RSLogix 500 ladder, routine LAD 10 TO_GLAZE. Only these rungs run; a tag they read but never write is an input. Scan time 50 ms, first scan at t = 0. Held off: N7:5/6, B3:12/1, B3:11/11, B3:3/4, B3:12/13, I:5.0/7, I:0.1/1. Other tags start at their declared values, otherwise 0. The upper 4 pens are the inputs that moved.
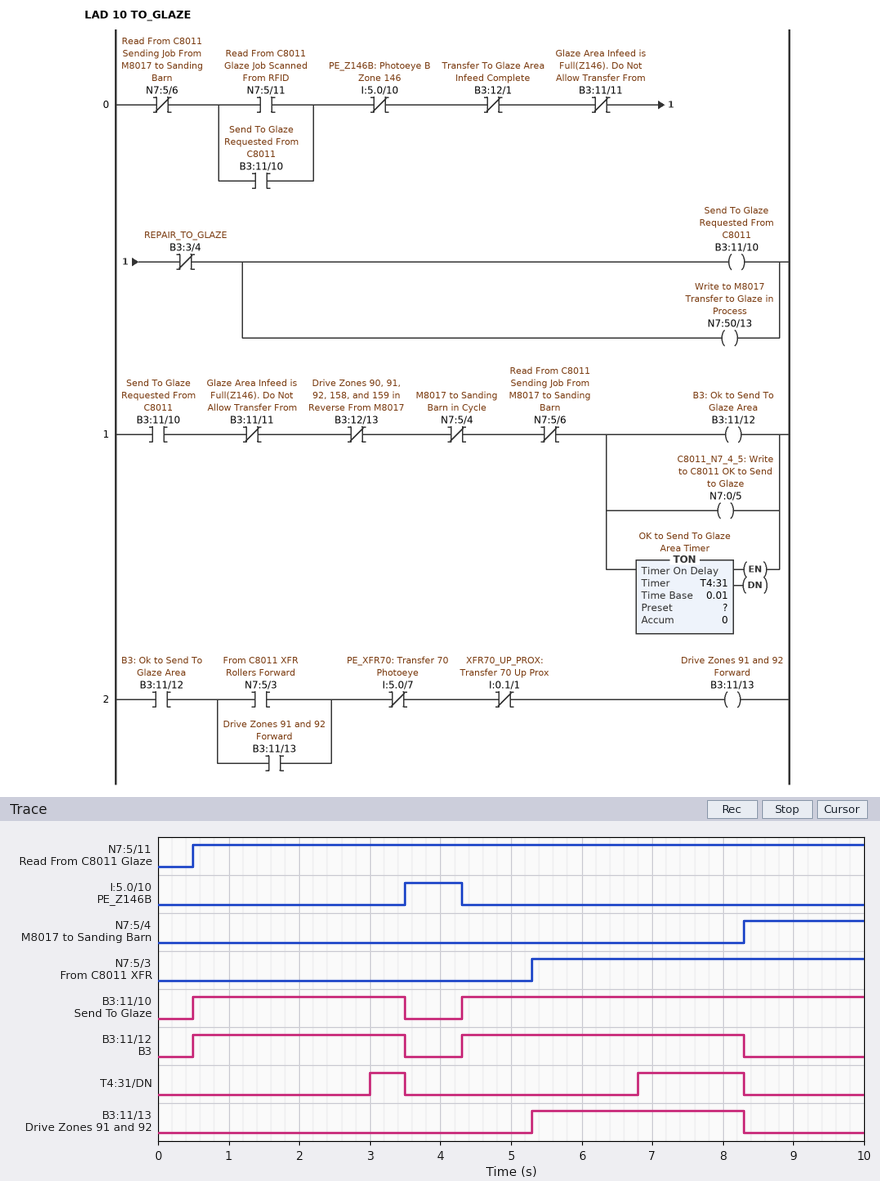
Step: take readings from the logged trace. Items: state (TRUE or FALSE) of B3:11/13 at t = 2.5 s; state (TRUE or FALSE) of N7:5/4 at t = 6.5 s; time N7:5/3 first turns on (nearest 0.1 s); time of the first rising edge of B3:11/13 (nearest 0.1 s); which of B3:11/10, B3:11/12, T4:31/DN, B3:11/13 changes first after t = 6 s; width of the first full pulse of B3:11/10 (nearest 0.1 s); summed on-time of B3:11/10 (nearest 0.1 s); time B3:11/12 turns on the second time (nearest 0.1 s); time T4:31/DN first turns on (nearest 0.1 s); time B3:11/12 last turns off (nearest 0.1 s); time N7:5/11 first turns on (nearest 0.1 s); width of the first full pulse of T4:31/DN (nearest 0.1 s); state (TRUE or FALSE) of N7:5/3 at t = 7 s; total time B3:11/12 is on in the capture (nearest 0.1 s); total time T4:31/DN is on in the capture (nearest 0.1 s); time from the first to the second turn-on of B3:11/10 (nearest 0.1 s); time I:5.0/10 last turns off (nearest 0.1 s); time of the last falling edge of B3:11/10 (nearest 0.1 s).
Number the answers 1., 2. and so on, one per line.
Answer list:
1. FALSE
2. FALSE
3. 5.3 s
4. 5.3 s
5. T4:31/DN
6. 3.0 s
7. 8.7 s
8. 4.3 s
9. 3.0 s
10. 8.3 s
11. 0.5 s
12. 0.5 s
13. TRUE
14. 7.0 s
15. 2.0 s
16. 3.8 s
17. 4.3 s
18. 3.5 s
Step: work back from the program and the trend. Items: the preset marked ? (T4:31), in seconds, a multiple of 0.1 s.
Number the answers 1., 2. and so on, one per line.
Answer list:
1. 2.5 s
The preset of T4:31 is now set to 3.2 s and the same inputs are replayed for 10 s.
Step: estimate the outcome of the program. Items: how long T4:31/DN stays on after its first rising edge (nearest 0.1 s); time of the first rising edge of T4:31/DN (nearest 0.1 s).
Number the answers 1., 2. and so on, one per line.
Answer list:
1. 0.8 s
2. 7.5 s
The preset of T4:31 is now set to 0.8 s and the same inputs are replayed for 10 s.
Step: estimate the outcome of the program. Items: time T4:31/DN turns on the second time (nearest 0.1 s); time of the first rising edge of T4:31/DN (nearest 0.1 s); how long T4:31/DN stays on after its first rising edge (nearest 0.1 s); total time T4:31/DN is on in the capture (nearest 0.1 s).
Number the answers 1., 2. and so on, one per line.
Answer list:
1. 5.1 s
2. 1.3 s
3. 2.2 s
4. 5.4 s
